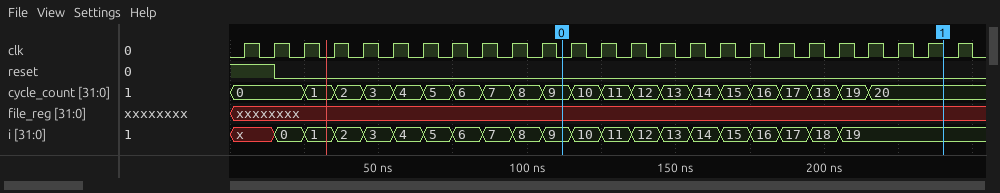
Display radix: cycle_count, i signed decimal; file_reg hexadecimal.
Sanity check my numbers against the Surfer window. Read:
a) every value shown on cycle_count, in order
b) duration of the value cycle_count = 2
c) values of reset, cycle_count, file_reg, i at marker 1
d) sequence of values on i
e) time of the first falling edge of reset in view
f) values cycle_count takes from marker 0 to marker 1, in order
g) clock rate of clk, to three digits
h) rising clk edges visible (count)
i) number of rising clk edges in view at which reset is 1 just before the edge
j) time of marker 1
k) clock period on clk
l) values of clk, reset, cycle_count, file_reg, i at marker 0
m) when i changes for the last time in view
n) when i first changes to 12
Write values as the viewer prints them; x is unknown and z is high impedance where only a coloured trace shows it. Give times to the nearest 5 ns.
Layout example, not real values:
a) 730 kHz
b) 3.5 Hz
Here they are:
a) 0, 1, 2, 3, 4, 5, 6, 7, 8, 9, 10, 11, 12, 13, 14, 15, 16, 17, 18, 19, 20
b) 10 ns
c) reset=0, cycle_count=20, file_reg=xxxxxxxx, i=19
d) x, 0, 1, 2, 3, 4, 5, 6, 7, 8, 9, 10, 11, 12, 13, 14, 15, 16, 17, 18, 19
e) 15 ns
f) 9, 10, 11, 12, 13, 14, 15, 16, 17, 18, 19, 20
g) 100 MHz
h) 25
i) 2
j) 240 ns
k) 10 ns
l) clk=0, reset=0, cycle_count=9, file_reg=xxxxxxxx, i=9
m) 205 ns
n) 135 ns
